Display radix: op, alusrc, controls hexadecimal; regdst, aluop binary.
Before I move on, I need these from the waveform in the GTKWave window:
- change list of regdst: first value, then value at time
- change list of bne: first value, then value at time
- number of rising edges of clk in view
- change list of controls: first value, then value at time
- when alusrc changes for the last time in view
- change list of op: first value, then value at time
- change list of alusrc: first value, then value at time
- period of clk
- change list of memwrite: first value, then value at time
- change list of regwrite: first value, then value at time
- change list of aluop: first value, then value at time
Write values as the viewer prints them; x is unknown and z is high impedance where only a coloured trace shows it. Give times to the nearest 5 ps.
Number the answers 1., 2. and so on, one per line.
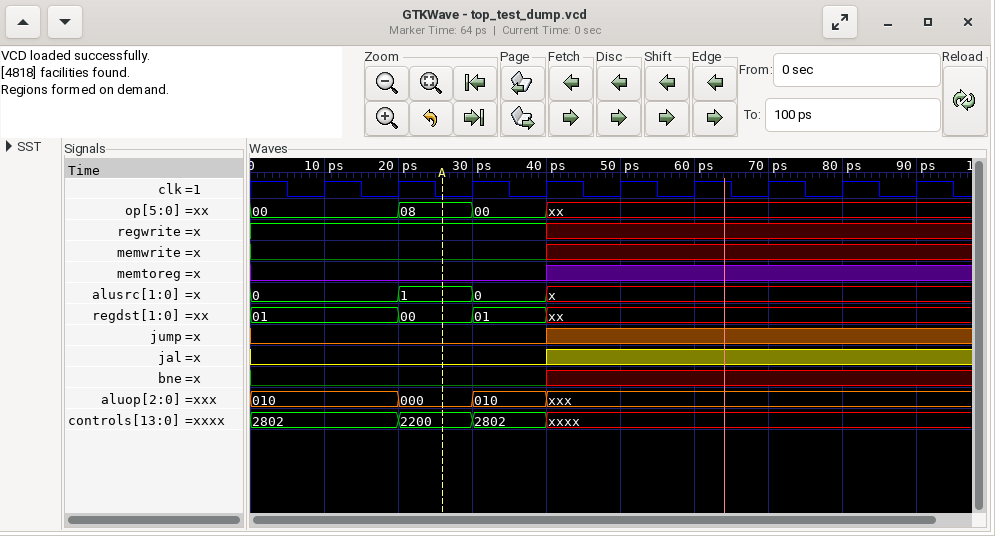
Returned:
1. 01, 00 at 20 ps, 01 at 30 ps, xx at 40 ps
2. 0, x at 40 ps
3. 9
4. 2802, 2200 at 20 ps, 2802 at 30 ps, xxxx at 40 ps
5. 40 ps
6. 00, 08 at 20 ps, 00 at 30 ps, xx at 40 ps
7. 0, 1 at 20 ps, 0 at 30 ps, x at 40 ps
8. 10 ps
9. 0, x at 40 ps
10. 1, x at 40 ps
11. 010, 000 at 20 ps, 010 at 30 ps, xxx at 40 ps
